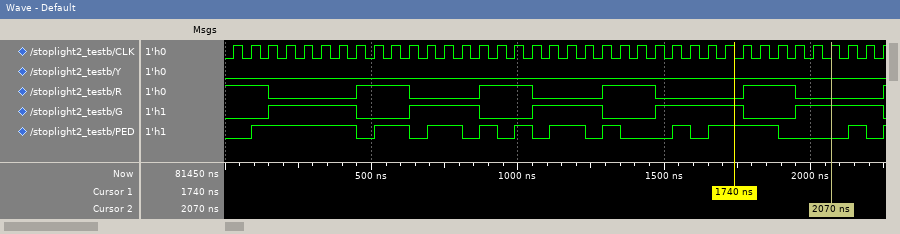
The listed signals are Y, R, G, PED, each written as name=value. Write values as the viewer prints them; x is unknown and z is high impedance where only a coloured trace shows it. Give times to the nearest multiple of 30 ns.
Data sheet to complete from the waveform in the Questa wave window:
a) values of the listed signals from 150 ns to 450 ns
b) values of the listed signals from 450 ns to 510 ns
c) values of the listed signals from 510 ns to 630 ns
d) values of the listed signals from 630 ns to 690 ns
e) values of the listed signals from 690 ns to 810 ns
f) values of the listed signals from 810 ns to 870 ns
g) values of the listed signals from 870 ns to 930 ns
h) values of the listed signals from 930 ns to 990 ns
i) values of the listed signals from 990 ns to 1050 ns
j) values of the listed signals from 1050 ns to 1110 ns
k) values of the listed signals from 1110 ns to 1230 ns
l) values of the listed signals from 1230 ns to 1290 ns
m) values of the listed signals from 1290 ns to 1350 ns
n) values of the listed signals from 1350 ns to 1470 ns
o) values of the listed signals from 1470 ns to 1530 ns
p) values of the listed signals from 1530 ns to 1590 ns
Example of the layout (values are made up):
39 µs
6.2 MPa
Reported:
Y=0, R=0, G=1, PED=1
Y=0, R=1, G=0, PED=0
Y=0, R=1, G=0, PED=1
Y=0, R=0, G=1, PED=0
Y=0, R=0, G=1, PED=1
Y=0, R=0, G=1, PED=0
Y=0, R=1, G=0, PED=1
Y=0, R=1, G=0, PED=0
Y=0, R=1, G=0, PED=1
Y=0, R=0, G=1, PED=0
Y=0, R=0, G=1, PED=1
Y=0, R=0, G=1, PED=0
Y=0, R=1, G=0, PED=1
Y=0, R=1, G=0, PED=0
Y=0, R=0, G=1, PED=0
Y=0, R=0, G=1, PED=1
